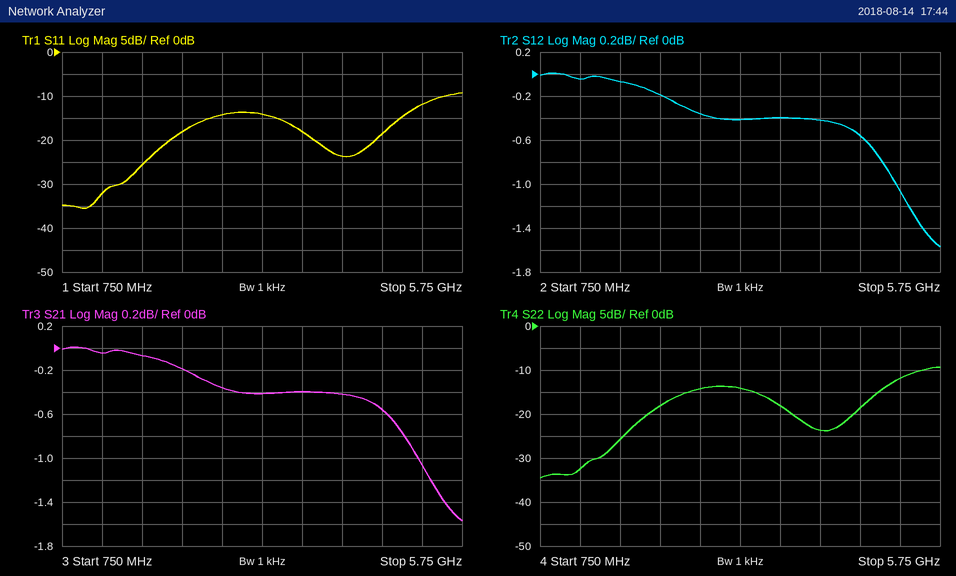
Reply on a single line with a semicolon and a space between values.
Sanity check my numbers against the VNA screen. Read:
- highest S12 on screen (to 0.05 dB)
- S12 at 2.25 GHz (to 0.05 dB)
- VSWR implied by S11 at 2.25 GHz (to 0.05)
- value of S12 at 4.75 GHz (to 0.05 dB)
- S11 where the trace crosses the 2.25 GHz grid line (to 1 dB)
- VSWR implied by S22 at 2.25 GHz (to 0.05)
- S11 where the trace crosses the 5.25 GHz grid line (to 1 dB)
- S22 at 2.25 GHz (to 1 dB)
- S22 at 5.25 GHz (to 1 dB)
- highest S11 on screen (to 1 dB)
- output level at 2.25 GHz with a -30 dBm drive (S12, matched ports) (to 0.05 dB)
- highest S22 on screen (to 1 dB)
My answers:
0.00 dB; -0.20 dB; 1.30; -0.55 dB; -18 dB; 1.30; -12 dB; -18 dB; -12 dB; -9 dB; -30.20 dBm; -9 dB
